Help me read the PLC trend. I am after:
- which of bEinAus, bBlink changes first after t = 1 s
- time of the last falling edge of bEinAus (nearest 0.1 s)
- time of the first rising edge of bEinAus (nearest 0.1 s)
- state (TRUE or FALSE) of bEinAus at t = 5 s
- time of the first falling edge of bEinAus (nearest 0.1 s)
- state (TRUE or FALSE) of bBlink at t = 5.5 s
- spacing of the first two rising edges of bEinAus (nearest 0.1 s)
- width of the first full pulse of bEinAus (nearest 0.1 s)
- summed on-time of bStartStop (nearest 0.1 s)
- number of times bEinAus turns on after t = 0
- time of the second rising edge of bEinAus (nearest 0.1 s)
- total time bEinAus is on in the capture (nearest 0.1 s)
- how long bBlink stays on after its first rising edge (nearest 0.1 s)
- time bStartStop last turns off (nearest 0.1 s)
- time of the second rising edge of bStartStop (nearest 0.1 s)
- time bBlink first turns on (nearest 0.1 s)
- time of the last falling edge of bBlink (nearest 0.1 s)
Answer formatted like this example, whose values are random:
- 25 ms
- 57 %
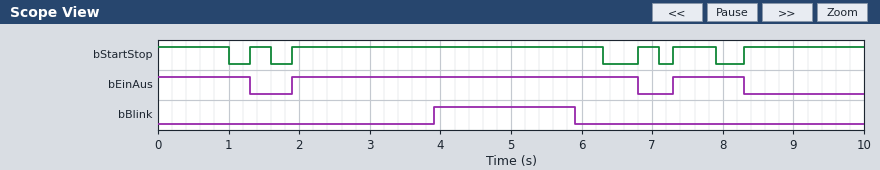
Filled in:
- bEinAus
- 8.3 s
- 1.9 s
- TRUE
- 1.3 s
- TRUE
- 5.4 s
- 4.9 s
- 8.3 s
- 2
- 7.3 s
- 7.2 s
- 2.0 s
- 7.9 s
- 1.9 s
- 3.9 s
- 5.9 s
